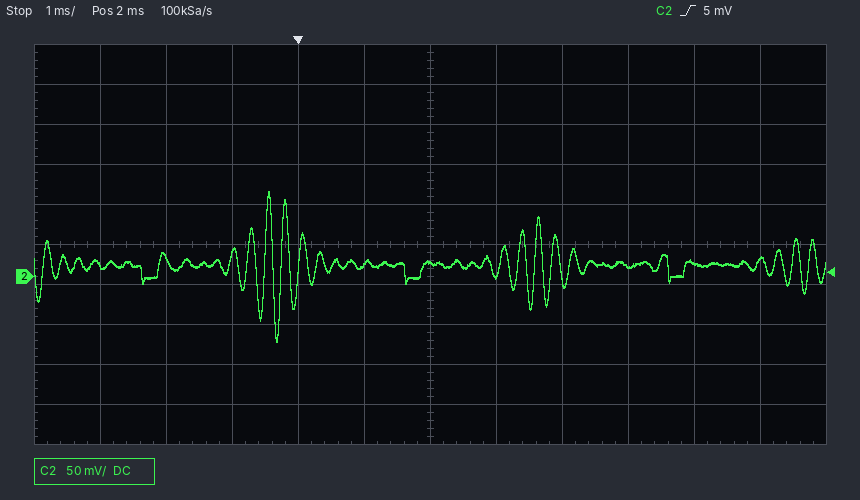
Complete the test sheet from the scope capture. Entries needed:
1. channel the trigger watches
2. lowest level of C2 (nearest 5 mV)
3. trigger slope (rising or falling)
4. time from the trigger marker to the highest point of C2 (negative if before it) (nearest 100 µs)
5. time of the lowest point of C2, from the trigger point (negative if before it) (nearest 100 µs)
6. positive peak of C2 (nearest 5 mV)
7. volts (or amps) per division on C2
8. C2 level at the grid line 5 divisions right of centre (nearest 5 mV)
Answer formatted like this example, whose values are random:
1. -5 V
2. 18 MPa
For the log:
1. C2
2. -80 mV
3. rising
4. -400 µs
5. -300 µs
6. 105 mV
7. 50 mV
8. 20 mV
